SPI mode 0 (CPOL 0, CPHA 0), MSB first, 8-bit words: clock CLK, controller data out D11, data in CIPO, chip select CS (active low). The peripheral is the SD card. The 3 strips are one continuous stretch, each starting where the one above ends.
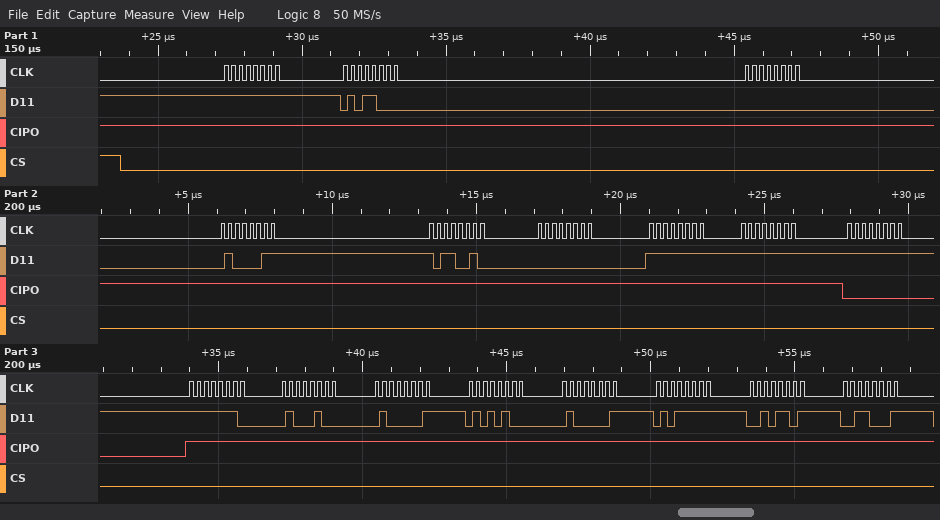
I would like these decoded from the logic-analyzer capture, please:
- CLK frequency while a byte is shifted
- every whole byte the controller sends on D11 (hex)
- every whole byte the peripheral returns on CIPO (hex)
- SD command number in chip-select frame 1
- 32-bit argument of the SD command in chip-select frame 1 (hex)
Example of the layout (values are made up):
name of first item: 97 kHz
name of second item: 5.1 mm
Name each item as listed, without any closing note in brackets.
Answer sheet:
CLK frequency while a byte is shifted: 4 MHz
every whole byte the controller sends on D11: FF 58 00 43 B2 00 FF FF FF FE 44 41 54 41 5F 2D 31
every whole byte the peripheral returns on CIPO: FF FF FF FF FF FF FF FF 00 FF FF FF FF FF FF FF FF
SD command number in chip-select frame 1: CMD24
32-bit argument of the SD command in chip-select frame 1: 0x0043B200
